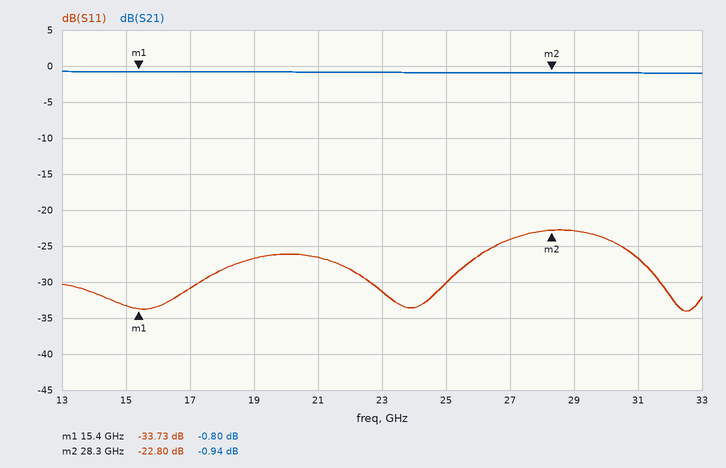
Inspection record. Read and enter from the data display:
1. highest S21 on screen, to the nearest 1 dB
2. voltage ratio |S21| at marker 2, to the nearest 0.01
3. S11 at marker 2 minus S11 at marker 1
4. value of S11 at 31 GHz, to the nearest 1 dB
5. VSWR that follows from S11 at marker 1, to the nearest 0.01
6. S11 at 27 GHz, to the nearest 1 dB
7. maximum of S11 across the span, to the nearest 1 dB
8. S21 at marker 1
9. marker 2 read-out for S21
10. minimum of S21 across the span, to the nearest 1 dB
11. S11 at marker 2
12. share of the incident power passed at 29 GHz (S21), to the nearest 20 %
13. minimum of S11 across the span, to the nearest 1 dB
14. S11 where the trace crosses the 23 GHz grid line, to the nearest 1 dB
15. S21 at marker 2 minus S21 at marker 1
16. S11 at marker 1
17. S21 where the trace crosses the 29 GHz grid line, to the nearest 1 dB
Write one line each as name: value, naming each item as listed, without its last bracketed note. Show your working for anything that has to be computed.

highest S21 on screen, to the nearest 1 dB: -1 dB
voltage ratio |S21| at marker 2, to the nearest 0.01: 10^(-0.94/20) ≈ 0.90
S11 at marker 2 minus S11 at marker 1: -22.8 − (-33.73) = 10.93 dB
value of S11 at 31 GHz, to the nearest 1 dB: -27 dB
VSWR that follows from S11 at marker 1, to the nearest 0.01: (1 + 0.0206)/(1 − 0.0206) ≈ 1.04
S11 at 27 GHz, to the nearest 1 dB: -24 dB
maximum of S11 across the span, to the nearest 1 dB: -23 dB
S21 at marker 1: -0.80 dB
marker 2 read-out for S21: -0.94 dB
minimum of S21 across the span, to the nearest 1 dB: -1 dB
S11 at marker 2: -22.80 dB
share of the incident power passed at 29 GHz (S21), to the nearest 20 %: 10^(-1/10) ≈ 79.4 %, so 80 % to the nearest 20 %
minimum of S11 across the span, to the nearest 1 dB: -34 dB
S11 where the trace crosses the 23 GHz grid line, to the nearest 1 dB: -31 dB
S21 at marker 2 minus S21 at marker 1: -0.94 − (-0.8) = -0.14 dB
S11 at marker 1: -33.73 dB
S21 where the trace crosses the 29 GHz grid line, to the nearest 1 dB: -1 dB
